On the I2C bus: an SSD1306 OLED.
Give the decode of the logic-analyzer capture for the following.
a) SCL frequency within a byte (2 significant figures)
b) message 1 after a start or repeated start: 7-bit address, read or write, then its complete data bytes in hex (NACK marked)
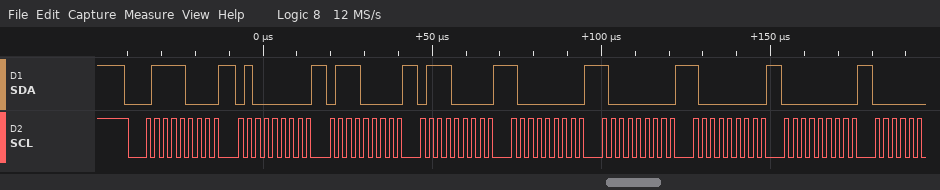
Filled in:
400 kHz
0x3C write: 40 70 70 80 80 80 00
